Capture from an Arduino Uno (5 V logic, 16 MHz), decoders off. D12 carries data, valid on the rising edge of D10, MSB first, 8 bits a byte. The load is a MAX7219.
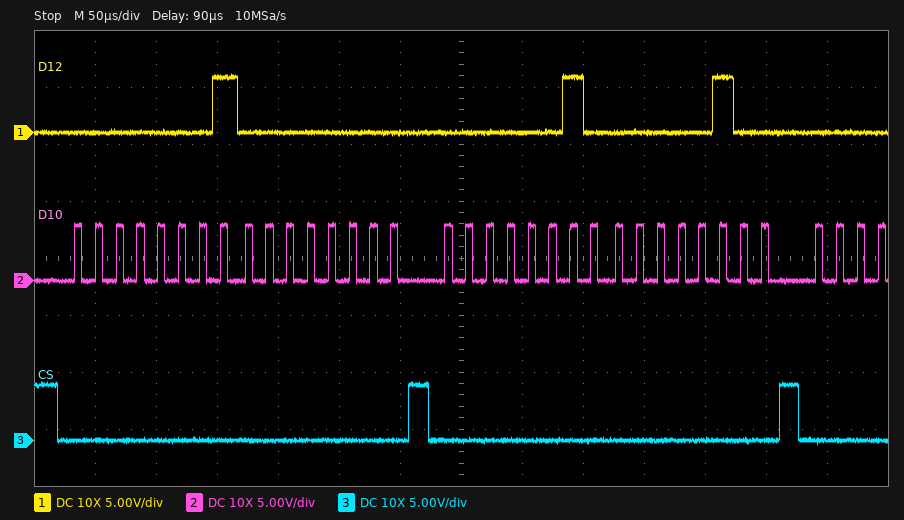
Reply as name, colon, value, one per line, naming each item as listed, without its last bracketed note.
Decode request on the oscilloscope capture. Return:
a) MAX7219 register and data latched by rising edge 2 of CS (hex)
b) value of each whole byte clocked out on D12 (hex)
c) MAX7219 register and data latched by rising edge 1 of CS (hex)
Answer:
MAX7219 register and data latched by rising edge 2 of CS: register 0x2, data 0x04
value of each whole byte clocked out on D12: 01 00 02 04
MAX7219 register and data latched by rising edge 1 of CS: register 0x1, data 0x00
